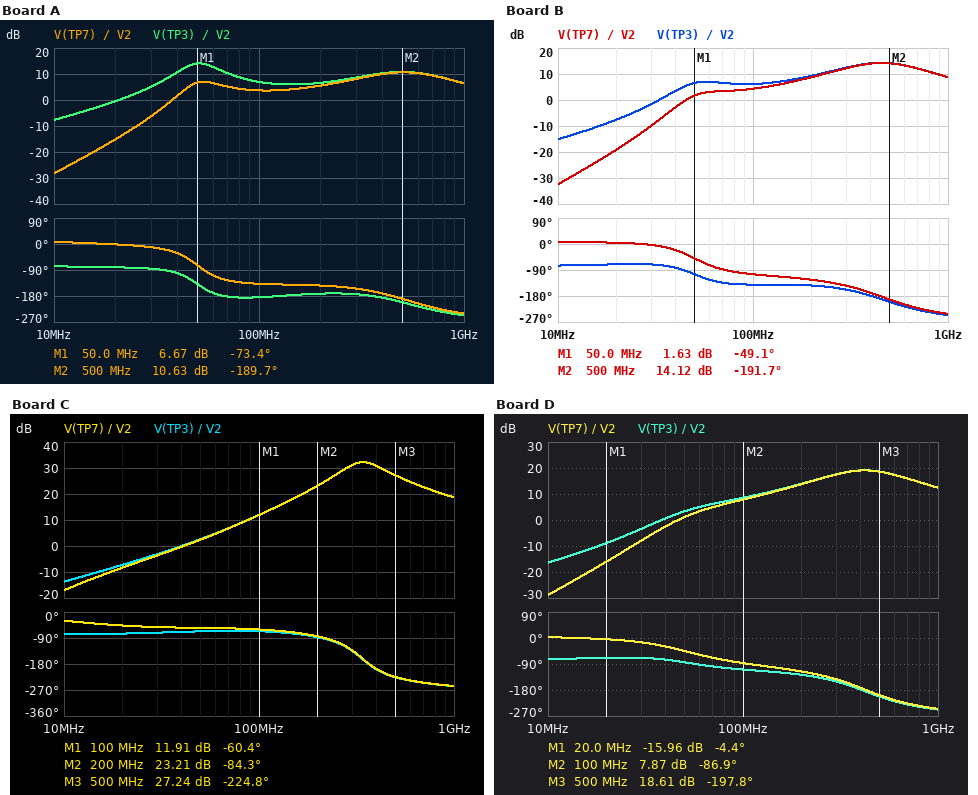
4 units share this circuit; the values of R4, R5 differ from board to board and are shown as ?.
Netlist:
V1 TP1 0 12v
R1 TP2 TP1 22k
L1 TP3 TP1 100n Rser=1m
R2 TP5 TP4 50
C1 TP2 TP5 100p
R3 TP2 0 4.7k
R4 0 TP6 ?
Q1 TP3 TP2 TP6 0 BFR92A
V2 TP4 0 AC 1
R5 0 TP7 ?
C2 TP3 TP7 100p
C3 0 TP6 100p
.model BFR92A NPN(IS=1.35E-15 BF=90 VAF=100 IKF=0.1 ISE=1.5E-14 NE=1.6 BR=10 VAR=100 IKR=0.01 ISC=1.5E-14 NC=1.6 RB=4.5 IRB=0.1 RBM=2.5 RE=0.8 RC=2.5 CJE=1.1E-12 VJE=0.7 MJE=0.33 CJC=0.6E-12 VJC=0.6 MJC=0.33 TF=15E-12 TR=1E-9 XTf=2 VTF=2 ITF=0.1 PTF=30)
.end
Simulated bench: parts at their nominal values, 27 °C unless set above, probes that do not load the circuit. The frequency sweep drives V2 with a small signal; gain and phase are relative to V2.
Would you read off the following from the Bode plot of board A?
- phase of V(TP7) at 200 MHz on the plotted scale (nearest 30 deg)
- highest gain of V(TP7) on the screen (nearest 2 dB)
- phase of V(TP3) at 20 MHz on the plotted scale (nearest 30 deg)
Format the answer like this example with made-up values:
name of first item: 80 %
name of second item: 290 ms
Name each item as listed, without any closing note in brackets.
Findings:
phase of V(TP7) at 200 MHz on the plotted scale: -150 deg
highest gain of V(TP7) on the screen: 10 dB
phase of V(TP3) at 20 MHz on the plotted scale: -90 deg
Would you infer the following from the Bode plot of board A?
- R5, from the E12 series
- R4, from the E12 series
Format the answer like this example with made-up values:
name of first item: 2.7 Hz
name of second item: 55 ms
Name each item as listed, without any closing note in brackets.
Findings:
R5, from the E12 series: 15 Ω
R4, from the E12 series: 12 Ω
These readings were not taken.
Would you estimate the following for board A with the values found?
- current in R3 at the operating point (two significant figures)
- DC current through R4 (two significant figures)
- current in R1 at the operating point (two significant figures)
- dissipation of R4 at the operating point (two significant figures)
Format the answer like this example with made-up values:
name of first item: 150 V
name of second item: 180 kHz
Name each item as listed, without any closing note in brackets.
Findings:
current in R3 at the operating point: 230 µA
DC current through R4: 22 mA
current in R1 at the operating point: 500 µA
dissipation of R4 at the operating point: 5.9 mW
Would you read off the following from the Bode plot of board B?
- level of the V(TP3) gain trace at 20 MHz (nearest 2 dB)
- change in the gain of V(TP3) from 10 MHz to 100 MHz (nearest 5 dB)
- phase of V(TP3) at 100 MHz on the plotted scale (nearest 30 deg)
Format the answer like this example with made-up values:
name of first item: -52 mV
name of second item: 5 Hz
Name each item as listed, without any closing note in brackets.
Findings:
level of the V(TP3) gain trace at 20 MHz: -8 dB
change in the gain of V(TP3) from 10 MHz to 100 MHz: 20 dB
phase of V(TP3) at 100 MHz on the plotted scale: -150 deg
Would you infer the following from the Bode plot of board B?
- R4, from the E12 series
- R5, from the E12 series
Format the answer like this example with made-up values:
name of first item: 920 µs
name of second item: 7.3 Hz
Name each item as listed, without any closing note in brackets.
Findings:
R4, from the E12 series: 33 Ω
R5, from the E12 series: 22 Ω
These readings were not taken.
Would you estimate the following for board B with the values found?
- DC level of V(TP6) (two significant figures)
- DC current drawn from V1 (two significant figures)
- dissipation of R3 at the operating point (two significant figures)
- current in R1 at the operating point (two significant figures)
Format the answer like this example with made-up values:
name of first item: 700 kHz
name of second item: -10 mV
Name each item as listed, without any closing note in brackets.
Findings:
DC level of V(TP6): 560 mV
DC current drawn from V1: 17 mA
dissipation of R3 at the operating point: 390 µW
current in R1 at the operating point: 480 µA
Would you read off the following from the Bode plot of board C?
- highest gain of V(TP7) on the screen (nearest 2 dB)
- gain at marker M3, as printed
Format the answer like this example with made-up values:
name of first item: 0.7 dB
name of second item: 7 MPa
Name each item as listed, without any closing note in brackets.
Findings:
highest gain of V(TP7) on the screen: 32 dB
gain at marker M3, as printed: 27.24 dB
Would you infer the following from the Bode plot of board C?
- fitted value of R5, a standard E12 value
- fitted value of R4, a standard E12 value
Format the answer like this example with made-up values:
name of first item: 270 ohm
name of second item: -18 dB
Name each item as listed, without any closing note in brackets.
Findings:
fitted value of R5, a standard E12 value: 150 Ω
fitted value of R4, a standard E12 value: 27 Ω
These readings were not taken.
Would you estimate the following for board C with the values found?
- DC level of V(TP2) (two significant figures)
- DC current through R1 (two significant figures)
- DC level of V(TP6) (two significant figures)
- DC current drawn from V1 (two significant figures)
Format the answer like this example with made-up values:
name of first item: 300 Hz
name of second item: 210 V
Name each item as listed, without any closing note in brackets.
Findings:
DC level of V(TP2): 1.3 V
DC current through R1: 490 µA
DC level of V(TP6): 490 mV
DC current drawn from V1: 18 mA
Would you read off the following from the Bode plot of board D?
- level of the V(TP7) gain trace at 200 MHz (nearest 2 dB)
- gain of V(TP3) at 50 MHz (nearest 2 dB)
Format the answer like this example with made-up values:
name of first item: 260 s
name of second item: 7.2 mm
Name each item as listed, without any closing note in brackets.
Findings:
level of the V(TP7) gain trace at 200 MHz: 14 dB
gain of V(TP3) at 50 MHz: 4 dB
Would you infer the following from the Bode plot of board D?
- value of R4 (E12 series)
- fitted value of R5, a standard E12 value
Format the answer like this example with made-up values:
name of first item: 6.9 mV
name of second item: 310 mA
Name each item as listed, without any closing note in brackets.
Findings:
value of R4: 39 Ω
fitted value of R5, a standard E12 value: 39 Ω
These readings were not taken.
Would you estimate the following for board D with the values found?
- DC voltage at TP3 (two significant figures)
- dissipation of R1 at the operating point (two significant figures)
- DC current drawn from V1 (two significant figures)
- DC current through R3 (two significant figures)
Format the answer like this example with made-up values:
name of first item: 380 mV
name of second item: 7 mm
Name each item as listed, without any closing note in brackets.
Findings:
DC voltage at TP3: 12 V
dissipation of R1 at the operating point: 5.1 mW
DC current drawn from V1: 16 mA
DC current through R3: 300 µA
